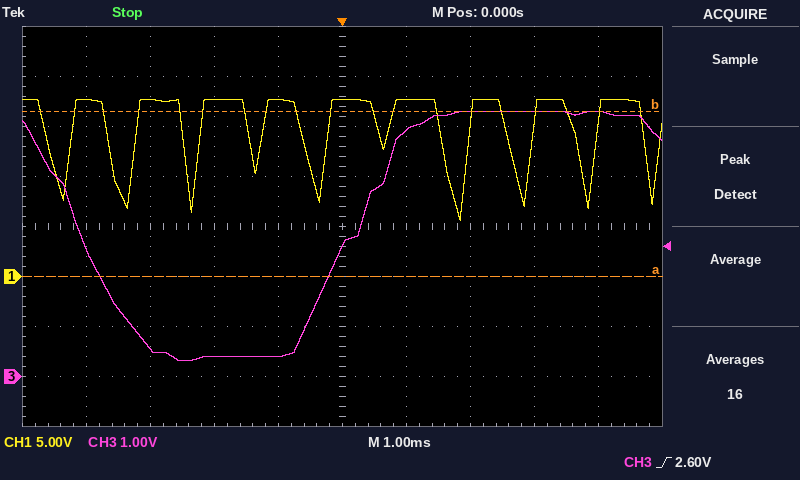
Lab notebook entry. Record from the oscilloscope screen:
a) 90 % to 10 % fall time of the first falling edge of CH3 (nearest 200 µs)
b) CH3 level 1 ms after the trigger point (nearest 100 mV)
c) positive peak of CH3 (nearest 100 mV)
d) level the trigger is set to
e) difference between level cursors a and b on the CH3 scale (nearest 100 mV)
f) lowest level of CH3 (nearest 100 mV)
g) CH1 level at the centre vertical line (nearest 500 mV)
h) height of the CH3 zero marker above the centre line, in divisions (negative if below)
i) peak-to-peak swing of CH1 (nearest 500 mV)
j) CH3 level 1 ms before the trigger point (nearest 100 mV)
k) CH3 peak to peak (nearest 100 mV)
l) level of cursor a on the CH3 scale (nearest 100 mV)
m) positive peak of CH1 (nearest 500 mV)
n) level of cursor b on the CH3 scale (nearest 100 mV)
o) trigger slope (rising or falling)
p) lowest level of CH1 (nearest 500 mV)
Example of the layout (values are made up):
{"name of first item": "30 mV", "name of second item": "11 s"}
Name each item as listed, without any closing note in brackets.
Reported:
{"90 % to 10 % fall time of the first falling edge of CH3": "1.6 ms", "CH3 level 1 ms after the trigger point": "4.9 V", "positive peak of CH3": "5.3 V", "level the trigger is set to": "2.60 V", "difference between level cursors a and b on the CH3 scale": "3.3 V", "lowest level of CH3": "300 mV", "CH1 level at the centre vertical line": "17.5 V", "height of the CH3 zero marker above the centre line, in divisions": "-3.0 div", "peak-to-peak swing of CH1": "12.0 V", "CH3 level 1 ms before the trigger point": "400 mV", "CH3 peak to peak": "5.0 V", "level of cursor a on the CH3 scale": "2.0 V", "positive peak of CH1": "17.5 V", "level of cursor b on the CH3 scale": "5.3 V", "trigger slope": "rising", "lowest level of CH1": "5.5 V"}
